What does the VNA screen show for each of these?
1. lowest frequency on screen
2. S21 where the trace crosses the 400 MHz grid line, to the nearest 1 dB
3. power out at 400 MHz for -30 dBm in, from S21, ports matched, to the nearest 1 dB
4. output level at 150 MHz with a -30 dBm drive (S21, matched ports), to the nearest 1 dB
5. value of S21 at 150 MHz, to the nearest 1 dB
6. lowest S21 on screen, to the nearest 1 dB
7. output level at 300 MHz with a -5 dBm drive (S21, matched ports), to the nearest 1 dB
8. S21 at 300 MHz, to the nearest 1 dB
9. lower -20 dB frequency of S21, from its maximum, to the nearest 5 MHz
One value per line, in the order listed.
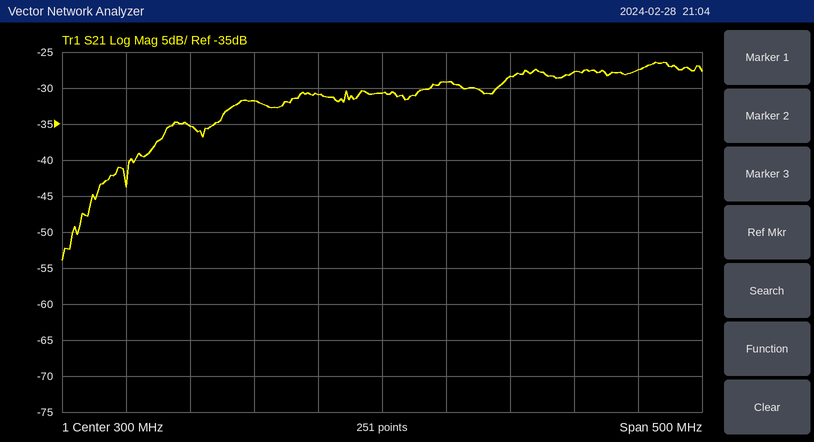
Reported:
50 MHz
-28 dB
-58 dBm
-65 dBm
-35 dB
-54 dB
-36 dBm
-31 dB
70 MHz
